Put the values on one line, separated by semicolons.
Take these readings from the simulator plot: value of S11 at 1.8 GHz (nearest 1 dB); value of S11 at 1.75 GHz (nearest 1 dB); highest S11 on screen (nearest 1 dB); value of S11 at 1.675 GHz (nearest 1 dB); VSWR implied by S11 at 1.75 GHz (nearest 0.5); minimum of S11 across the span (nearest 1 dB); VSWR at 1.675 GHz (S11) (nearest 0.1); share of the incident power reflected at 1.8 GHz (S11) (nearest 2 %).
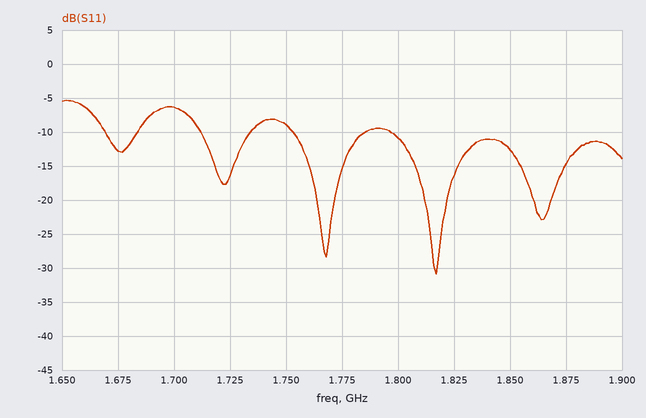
-11 dB; -9 dB; -5 dB; -13 dB; 2.0; -31 dB; 1.6; 8 %
